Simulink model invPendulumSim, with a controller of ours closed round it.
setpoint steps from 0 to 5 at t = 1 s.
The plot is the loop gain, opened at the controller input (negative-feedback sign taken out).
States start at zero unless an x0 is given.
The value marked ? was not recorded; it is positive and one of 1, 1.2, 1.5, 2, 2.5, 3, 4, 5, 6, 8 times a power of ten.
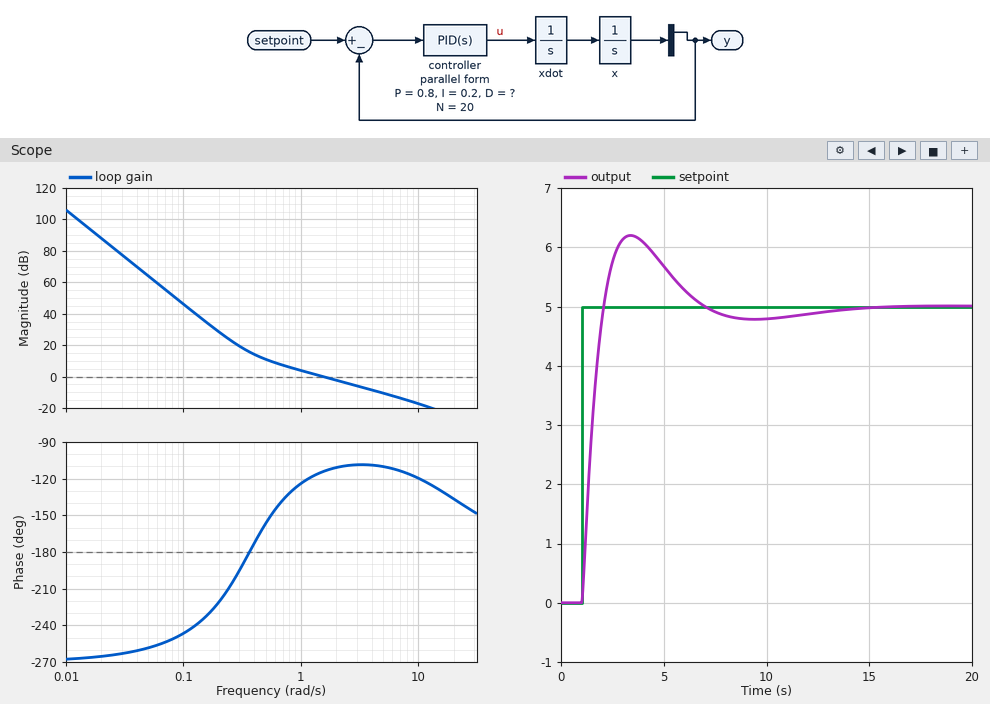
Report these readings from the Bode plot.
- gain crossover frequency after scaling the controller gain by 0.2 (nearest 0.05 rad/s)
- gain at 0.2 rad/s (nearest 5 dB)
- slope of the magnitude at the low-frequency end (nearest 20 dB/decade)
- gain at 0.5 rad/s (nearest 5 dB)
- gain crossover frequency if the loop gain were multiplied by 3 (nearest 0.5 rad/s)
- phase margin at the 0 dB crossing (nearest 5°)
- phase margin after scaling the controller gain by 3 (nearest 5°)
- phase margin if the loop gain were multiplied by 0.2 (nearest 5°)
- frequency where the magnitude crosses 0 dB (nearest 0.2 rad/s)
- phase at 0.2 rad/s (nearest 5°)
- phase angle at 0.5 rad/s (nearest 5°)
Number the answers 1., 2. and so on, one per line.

1. 0.40 rad/s
2. 30 dB
3. -60 dB/decade
4. 10 dB
5. 4.5 rad/s
6. 65°
7. 70°
8. 10°
9. 1.6 rad/s
10. -220°
11. -155°
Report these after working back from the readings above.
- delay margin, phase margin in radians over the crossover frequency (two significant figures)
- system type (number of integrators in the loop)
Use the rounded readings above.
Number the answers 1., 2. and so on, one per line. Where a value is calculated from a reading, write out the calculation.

1. 65 × π / 180 / 1.6 = 0.71 s
2. 3
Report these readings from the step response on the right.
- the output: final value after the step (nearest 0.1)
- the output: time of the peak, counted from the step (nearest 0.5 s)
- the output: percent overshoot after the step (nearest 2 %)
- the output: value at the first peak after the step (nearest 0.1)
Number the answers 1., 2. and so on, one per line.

1. 5.0
2. 2.5 s
3. 24 %
4. 6.2
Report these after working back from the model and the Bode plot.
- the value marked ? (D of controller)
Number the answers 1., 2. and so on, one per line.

1. 1.5
